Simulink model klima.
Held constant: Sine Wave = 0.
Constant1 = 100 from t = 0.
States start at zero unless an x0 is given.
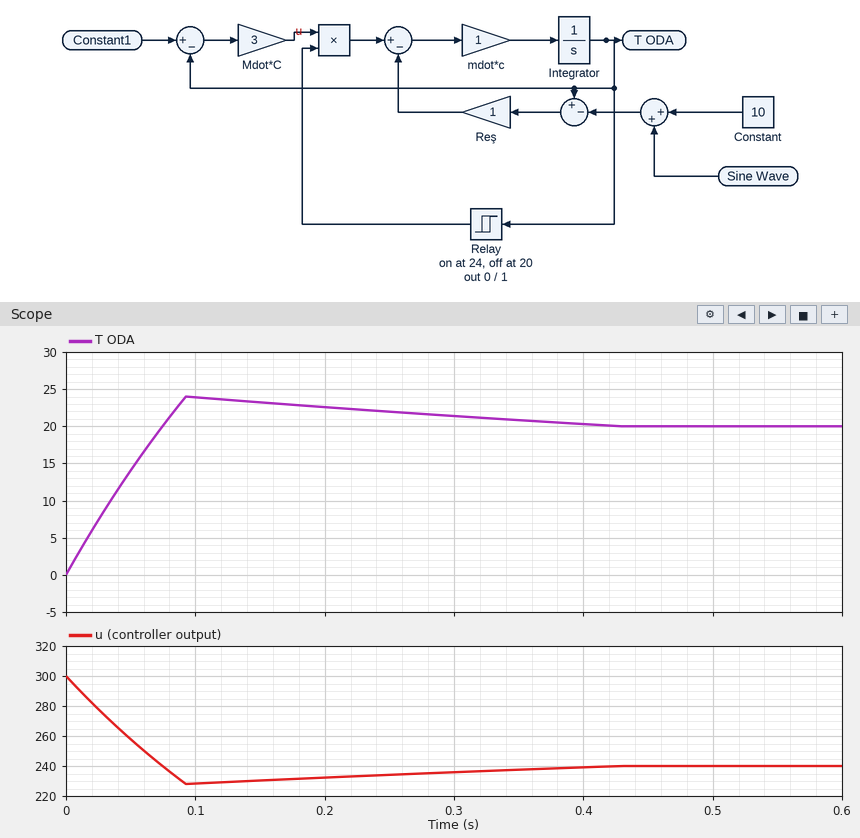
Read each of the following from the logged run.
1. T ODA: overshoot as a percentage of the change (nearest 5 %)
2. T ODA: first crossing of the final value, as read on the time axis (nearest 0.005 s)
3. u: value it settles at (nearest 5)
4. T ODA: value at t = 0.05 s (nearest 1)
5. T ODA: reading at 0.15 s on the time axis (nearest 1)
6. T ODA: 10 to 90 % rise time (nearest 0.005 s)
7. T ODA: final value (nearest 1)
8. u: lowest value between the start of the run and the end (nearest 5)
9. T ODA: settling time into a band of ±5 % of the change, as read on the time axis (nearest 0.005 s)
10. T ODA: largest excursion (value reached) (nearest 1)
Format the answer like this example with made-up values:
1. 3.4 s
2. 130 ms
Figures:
1. 20 %
2. 0.075 s
3. 240
4. 14
5. 23
6. 0.060 s
7. 20
8. 230
9. 0.330 s
10. 24
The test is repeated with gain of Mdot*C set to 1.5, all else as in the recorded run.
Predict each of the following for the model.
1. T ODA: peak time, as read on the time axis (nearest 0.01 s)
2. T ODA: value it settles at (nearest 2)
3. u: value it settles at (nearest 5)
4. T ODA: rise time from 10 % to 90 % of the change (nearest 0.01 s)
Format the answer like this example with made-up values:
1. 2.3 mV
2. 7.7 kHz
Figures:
1. 0.19 s
2. 20
3. 120
4. 0.12 s
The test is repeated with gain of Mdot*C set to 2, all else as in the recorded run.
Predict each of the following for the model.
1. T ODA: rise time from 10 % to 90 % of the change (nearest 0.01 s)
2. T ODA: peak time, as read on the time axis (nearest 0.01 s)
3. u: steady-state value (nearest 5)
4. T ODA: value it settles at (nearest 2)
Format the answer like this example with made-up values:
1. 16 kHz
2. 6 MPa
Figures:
1. 0.09 s
2. 0.14 s
3. 160
4. 20
